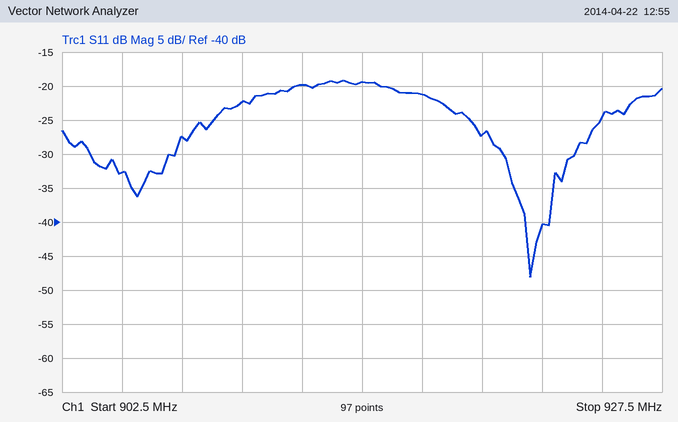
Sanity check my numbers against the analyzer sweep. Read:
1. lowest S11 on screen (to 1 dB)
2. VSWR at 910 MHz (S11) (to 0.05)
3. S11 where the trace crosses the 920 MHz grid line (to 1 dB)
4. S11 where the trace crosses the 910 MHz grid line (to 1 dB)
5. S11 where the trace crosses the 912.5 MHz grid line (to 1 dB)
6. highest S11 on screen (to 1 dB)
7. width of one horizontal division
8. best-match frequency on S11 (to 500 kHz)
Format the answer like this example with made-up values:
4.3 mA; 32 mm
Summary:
-48 dB; 1.15; -27 dB; -22 dB; -20 dB; -19 dB; 2.5 MHz; 922.0 MHz
